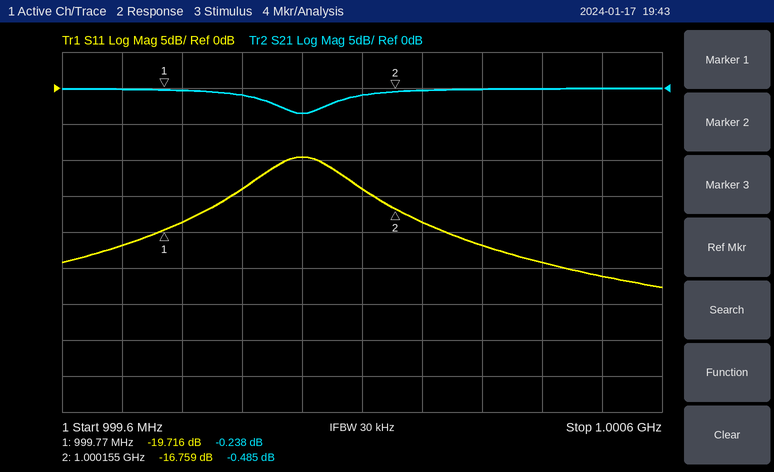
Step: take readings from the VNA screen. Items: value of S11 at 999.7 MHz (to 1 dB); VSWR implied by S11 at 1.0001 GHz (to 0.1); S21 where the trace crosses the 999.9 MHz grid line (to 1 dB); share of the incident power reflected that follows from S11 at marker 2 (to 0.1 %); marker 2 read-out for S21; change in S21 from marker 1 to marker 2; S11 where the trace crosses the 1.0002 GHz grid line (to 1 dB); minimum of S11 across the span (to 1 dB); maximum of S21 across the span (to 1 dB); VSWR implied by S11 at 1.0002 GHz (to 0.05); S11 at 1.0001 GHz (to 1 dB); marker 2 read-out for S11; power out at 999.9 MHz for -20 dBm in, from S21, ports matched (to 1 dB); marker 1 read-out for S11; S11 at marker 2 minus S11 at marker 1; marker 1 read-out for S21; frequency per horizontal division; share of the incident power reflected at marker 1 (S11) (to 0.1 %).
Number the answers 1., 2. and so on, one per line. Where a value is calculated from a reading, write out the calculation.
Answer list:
1. -22 dB
2. |Γ| = 10^(-14/20) = 0.1995; VSWR = (1 + 0.1995)/(1 − 0.1995) ≈ 1.5
3. -1 dB
4. 10^(-16.759/10) ≈ 2.1 %
5. -0.485 dB
6. -0.485 − (-0.238) = -0.247 dB
7. -19 dB
8. -28 dB
9. 0 dB
10. |Γ| = 10^(-19/20) = 0.1122; VSWR = (1 + 0.1122)/(1 − 0.1122) ≈ 1.25
11. -14 dB
12. -16.759 dB
13. -20 dBm + (-1 dB) = -21 dBm
14. -19.716 dB
15. -16.759 − (-19.716) = 2.957 dB
16. -0.238 dB
17. 100 kHz
18. 10^(-19.716/10) ≈ 1.1 %
